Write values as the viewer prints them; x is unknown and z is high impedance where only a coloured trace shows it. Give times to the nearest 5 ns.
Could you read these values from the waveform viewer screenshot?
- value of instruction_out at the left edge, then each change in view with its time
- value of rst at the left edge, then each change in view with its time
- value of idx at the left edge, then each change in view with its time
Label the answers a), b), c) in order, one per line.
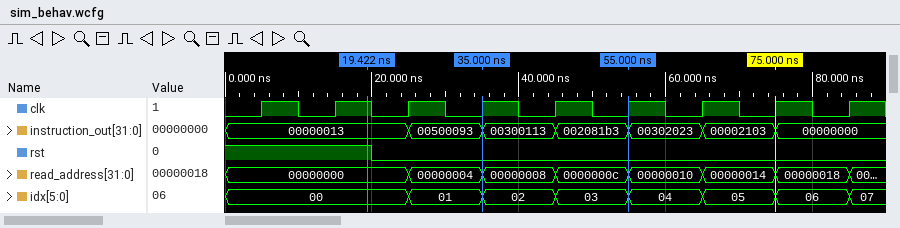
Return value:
a) 00000013, 00500093 at 25 ns, 00300113 at 35 ns, 002081b3 at 45 ns, 00302023 at 55 ns, 00002103 at 65 ns, 00000000 at 75 ns
b) 1, 0 at 20 ns
c) 00, 01 at 25 ns, 02 at 35 ns, 03 at 45 ns, 04 at 55 ns, 05 at 65 ns, 06 at 75 ns, 07 at 85 ns
